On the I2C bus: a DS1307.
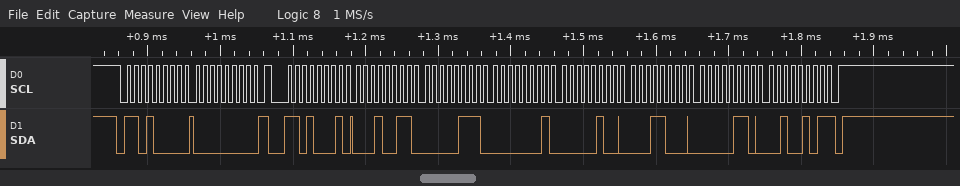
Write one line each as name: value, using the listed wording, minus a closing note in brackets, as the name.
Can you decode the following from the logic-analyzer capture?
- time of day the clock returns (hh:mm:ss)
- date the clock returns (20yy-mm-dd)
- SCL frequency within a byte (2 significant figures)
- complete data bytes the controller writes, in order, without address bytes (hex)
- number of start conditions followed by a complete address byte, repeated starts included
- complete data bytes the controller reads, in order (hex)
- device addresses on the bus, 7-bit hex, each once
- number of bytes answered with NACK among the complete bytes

time of day the clock returns: 01:07:13
date the clock returns: 2025-06-18
SCL frequency within a byte: 100 kHz
complete data bytes the controller writes, in order, without address bytes: 00
number of start conditions followed by a complete address byte, repeated starts included: 2
complete data bytes the controller reads, in order: 13 07 01 04 18 06 25
device addresses on the bus, 7-bit hex, each once: 0x68
number of bytes answered with NACK among the complete bytes: 1
